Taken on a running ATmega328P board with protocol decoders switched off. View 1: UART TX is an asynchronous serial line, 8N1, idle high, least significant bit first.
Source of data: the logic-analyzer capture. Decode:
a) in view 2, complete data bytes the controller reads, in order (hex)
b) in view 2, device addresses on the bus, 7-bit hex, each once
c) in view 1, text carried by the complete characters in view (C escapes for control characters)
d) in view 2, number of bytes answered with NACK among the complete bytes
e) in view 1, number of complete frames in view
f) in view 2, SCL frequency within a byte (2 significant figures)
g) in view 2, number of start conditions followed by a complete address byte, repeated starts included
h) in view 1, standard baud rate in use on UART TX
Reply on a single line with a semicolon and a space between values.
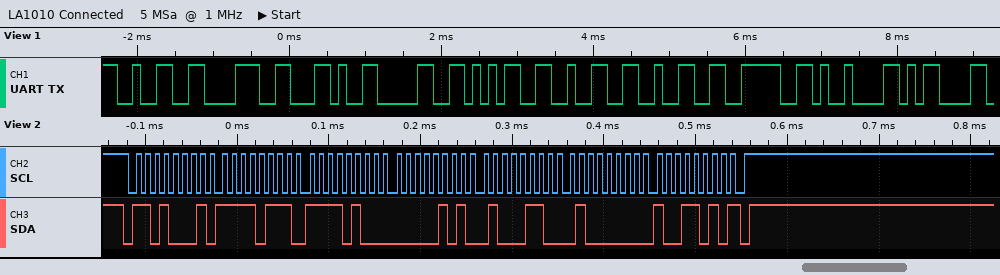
F7 F4 05 46 40 9A; 0x68; "28,0522>\t\r"; 1; 10; 100 kHz; 1; 9600 baud
